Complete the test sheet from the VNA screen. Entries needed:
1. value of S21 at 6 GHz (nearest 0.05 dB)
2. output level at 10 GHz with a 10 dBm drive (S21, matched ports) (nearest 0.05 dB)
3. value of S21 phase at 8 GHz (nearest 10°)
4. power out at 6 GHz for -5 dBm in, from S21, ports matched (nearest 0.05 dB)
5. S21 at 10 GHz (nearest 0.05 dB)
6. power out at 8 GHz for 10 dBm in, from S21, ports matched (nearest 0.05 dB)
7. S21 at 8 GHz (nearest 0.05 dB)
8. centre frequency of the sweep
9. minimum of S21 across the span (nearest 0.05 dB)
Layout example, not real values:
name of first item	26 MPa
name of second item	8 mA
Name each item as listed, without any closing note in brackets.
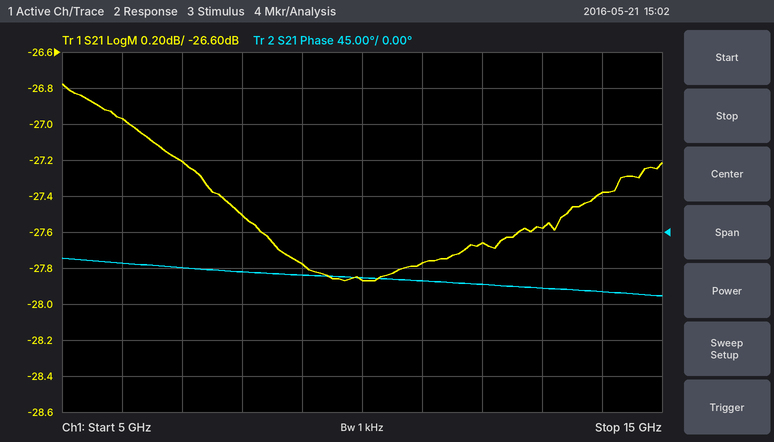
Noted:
value of S21 at 6 GHz	-26.95 dB
output level at 10 GHz with a 10 dBm drive (S21, matched ports)	-17.85 dBm
value of S21 phase at 8 GHz	-50°
power out at 6 GHz for -5 dBm in, from S21, ports matched	-31.95 dBm
S21 at 10 GHz	-27.85 dB
power out at 8 GHz for 10 dBm in, from S21, ports matched	-17.50 dBm
S21 at 8 GHz	-27.50 dB
centre frequency of the sweep	10 GHz
minimum of S21 across the span	-27.85 dB
